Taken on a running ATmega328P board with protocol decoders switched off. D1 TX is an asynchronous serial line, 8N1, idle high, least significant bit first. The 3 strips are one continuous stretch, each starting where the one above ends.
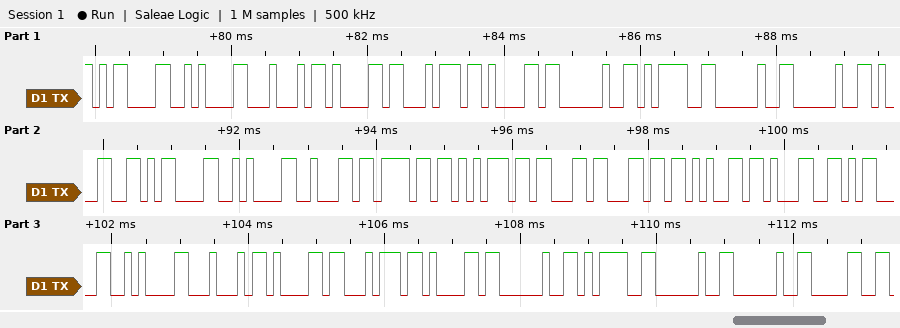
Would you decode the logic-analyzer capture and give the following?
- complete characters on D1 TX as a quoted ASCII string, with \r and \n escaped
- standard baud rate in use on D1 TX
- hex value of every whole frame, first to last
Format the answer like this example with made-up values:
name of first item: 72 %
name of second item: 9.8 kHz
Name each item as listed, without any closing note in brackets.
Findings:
complete characters on D1 TX as a quoted ASCII string, with \r and \n escaped: "\r\nData =  1\r\nboucle1\r\nData =  0"
standard baud rate in use on D1 TX: 9600 baud
hex value of every whole frame, first to last: 0D 0A 44 61 74 61 20 3D 20 20 31 0D 0A 62 6F 75 63 6C 65 31 0D 0A 44 61 74 61 20 3D 20 20 30
